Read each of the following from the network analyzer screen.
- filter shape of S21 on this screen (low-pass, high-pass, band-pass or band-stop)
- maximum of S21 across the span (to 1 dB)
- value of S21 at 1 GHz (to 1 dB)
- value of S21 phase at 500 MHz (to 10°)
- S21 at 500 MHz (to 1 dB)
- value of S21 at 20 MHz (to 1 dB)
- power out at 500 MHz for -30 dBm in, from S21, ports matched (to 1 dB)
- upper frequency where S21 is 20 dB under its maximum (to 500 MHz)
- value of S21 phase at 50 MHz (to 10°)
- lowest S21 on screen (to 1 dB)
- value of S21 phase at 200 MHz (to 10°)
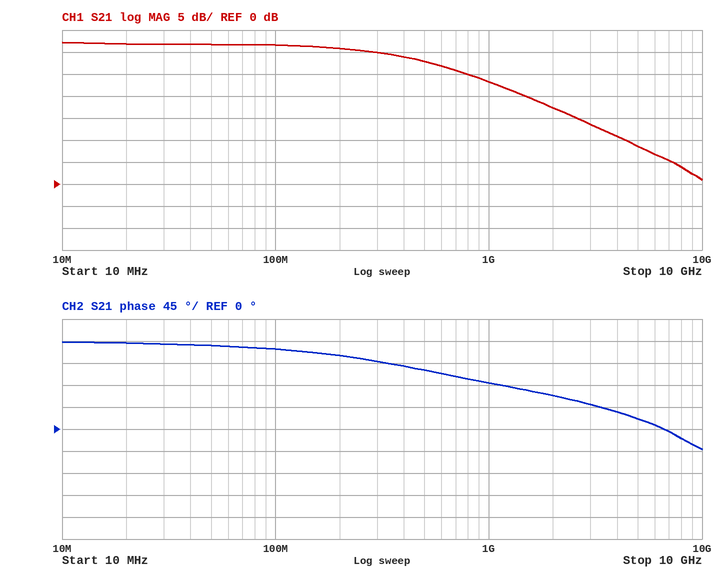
low-pass
32 dB
23 dB
120°
28 dB
32 dB
-2 dBm
3.5 GHz
170°
1 dB
150°
